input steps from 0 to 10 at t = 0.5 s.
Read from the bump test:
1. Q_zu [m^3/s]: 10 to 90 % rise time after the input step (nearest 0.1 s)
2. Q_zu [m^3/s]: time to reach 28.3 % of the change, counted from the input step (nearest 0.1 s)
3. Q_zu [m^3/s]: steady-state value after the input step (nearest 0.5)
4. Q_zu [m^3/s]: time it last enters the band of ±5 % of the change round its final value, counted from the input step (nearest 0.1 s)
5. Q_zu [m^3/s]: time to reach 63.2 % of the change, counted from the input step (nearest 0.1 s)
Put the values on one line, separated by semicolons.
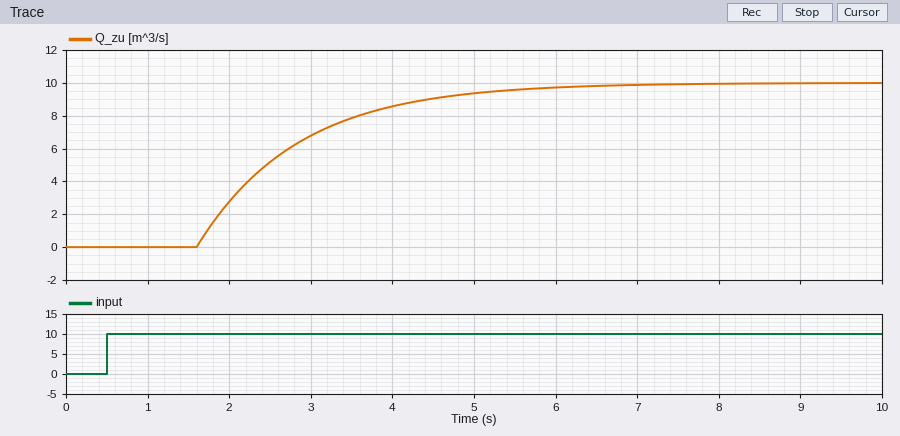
2.7 s; 1.5 s; 10.0; 4.8 s; 2.3 s
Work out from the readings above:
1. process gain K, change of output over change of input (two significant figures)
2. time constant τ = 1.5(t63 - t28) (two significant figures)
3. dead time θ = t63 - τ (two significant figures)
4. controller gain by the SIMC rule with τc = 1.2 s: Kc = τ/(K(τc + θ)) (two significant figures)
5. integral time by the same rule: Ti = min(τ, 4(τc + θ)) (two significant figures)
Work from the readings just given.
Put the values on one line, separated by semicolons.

1.0; 1.2 s; 1.1 s; 0.52; 1.2 s
